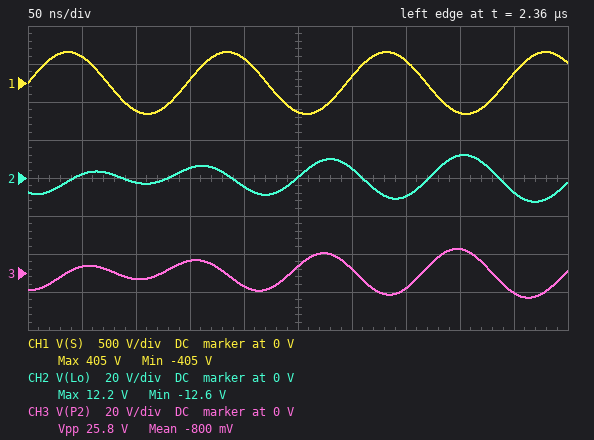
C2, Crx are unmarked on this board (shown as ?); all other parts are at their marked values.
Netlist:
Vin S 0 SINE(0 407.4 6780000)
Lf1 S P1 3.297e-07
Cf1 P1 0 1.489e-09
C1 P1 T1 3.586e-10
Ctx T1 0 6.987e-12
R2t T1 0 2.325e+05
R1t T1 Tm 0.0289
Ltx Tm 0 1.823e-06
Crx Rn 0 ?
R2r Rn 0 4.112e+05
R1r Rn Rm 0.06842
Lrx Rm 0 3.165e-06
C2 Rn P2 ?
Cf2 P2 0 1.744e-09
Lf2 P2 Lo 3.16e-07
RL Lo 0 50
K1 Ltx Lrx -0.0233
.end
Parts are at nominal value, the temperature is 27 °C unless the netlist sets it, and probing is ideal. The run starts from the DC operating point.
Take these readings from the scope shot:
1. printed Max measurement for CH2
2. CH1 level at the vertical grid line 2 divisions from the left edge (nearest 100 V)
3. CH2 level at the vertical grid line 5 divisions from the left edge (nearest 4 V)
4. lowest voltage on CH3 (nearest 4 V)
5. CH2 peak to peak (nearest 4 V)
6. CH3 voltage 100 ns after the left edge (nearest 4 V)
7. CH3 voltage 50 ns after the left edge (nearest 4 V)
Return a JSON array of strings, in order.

["12.2 V", "-400 V", "0 V", "-12 V", "24 V", "-4 V", "4 V"]
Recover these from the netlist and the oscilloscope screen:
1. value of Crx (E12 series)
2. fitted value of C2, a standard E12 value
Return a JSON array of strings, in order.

["12 pF", "82 pF"]
